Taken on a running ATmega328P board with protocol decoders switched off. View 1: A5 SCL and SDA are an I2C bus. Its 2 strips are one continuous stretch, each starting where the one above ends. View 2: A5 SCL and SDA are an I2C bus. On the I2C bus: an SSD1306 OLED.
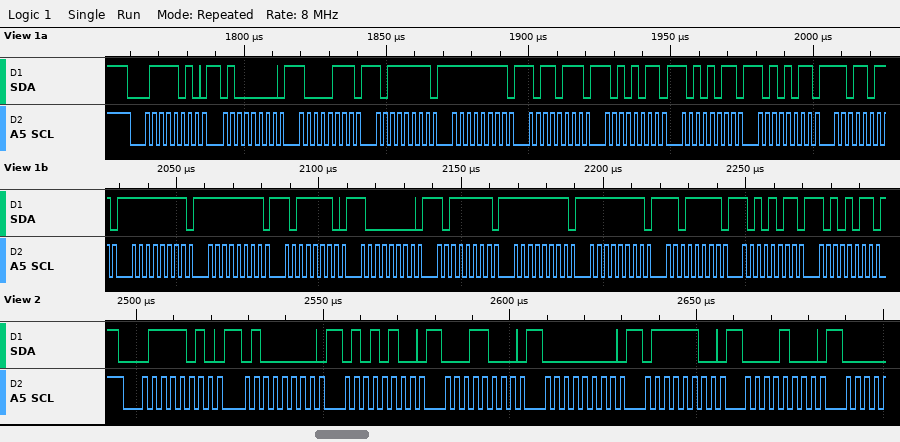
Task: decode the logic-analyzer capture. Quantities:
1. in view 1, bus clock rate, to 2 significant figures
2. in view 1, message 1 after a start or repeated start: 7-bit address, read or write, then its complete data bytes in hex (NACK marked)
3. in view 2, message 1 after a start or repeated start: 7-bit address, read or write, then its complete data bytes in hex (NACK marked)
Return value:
400 kHz
0x3D write: 40 87 BF FF B7 AB AB AB DB FF FF BE 80 BF FF FF DF AB AB
0x3D write: 40 54 18 00 7C 08
